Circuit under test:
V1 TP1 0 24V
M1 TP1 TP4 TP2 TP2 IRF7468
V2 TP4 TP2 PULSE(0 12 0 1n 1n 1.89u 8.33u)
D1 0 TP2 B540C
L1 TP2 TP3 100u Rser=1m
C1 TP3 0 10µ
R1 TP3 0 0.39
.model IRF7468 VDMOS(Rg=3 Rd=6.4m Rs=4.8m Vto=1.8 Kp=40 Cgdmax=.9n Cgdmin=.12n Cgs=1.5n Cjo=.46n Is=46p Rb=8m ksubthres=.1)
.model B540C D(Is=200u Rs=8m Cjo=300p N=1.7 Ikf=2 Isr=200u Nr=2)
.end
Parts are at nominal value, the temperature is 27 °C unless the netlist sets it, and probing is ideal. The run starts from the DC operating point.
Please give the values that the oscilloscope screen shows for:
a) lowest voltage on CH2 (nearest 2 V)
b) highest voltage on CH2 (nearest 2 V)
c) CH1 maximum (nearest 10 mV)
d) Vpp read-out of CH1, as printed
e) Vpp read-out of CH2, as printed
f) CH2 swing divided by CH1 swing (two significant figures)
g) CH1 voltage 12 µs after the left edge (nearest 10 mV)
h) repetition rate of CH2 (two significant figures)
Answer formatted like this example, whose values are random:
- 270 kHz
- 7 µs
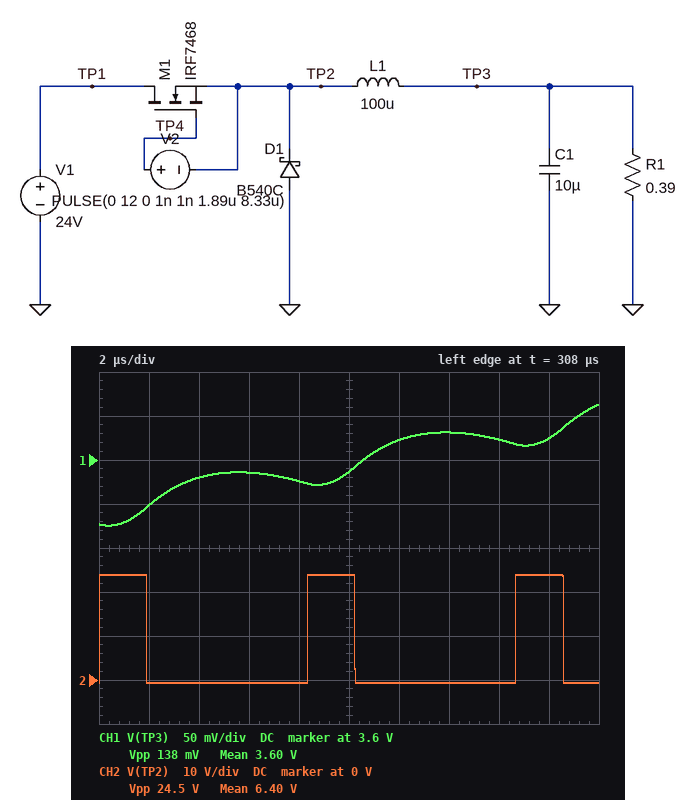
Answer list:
- 0 V
- 24 V
- 3.66 V
- 138 mV
- 24.5 V
- 180
- 3.62 V
- 120 kHz
